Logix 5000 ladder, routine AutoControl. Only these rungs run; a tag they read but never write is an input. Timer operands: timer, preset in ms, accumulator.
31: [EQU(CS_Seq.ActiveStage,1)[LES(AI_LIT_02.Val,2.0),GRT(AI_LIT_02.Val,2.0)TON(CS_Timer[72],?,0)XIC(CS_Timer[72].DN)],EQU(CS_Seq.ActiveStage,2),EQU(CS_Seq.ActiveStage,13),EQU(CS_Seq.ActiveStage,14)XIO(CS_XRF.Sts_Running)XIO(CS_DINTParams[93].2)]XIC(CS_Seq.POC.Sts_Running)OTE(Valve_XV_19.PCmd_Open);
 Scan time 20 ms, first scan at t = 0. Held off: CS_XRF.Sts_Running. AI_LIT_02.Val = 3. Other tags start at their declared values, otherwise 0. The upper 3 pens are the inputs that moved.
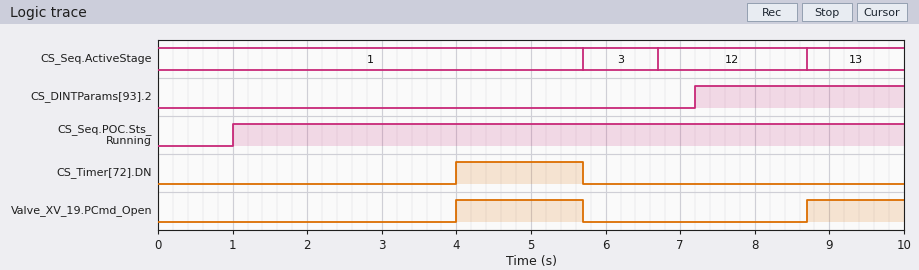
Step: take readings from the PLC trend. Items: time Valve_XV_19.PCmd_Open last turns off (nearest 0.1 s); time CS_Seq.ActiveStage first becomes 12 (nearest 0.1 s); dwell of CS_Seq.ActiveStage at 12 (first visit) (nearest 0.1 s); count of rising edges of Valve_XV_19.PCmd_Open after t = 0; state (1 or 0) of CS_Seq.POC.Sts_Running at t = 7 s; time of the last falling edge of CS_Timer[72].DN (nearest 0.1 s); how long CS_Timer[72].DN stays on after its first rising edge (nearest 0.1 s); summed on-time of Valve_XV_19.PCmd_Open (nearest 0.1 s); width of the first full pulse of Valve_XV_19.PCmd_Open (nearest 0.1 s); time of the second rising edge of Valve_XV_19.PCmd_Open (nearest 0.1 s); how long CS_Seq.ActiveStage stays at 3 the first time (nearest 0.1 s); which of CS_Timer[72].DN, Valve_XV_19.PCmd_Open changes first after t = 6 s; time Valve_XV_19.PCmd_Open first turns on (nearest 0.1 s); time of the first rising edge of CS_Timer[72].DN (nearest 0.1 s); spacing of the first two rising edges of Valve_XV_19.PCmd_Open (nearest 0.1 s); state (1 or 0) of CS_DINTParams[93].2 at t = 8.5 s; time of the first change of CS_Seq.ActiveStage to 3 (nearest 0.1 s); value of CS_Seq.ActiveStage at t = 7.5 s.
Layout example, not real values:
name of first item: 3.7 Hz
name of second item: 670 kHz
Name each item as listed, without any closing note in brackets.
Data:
time Valve_XV_19.PCmd_Open last turns off: 5.7 s
time CS_Seq.ActiveStage first becomes 12: 6.7 s
dwell of CS_Seq.ActiveStage at 12 (first visit): 2.0 s
count of rising edges of Valve_XV_19.PCmd_Open after t = 0: 2
state (1 or 0) of CS_Seq.POC.Sts_Running at t = 7 s: 1
time of the last falling edge of CS_Timer[72].DN: 5.7 s
how long CS_Timer[72].DN stays on after its first rising edge: 1.7 s
summed on-time of Valve_XV_19.PCmd_Open: 3.0 s
width of the first full pulse of Valve_XV_19.PCmd_Open: 1.7 s
time of the second rising edge of Valve_XV_19.PCmd_Open: 8.7 s
how long CS_Seq.ActiveStage stays at 3 the first time: 1.0 s
which of CS_Timer[72].DN, Valve_XV_19.PCmd_Open changes first after t = 6 s: Valve_XV_19.PCmd_Open
time Valve_XV_19.PCmd_Open first turns on: 4.0 s
time of the first rising edge of CS_Timer[72].DN: 4.0 s
spacing of the first two rising edges of Valve_XV_19.PCmd_Open: 4.7 s
state (1 or 0) of CS_DINTParams[93].2 at t = 8.5 s: 1
time of the first change of CS_Seq.ActiveStage to 3: 5.7 s
value of CS_Seq.ActiveStage at t = 7.5 s: 12
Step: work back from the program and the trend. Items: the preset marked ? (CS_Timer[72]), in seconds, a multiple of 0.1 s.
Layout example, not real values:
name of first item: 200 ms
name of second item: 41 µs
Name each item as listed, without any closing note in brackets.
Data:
the preset marked ? (CS_Timer[72]), in seconds, a multiple of 0.1 s: 4.0 s
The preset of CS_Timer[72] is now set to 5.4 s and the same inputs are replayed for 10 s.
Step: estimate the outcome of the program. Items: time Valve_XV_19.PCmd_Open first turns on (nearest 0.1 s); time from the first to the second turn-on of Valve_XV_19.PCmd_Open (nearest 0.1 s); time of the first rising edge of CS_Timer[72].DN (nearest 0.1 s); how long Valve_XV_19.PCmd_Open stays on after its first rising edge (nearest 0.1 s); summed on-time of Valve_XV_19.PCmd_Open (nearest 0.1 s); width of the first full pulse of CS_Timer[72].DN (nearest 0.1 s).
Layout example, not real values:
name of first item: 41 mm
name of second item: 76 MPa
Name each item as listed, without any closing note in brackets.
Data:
time Valve_XV_19.PCmd_Open first turns on: 5.4 s
time from the first to the second turn-on of Valve_XV_19.PCmd_Open: 3.3 s
time of the first rising edge of CS_Timer[72].DN: 5.4 s
how long Valve_XV_19.PCmd_Open stays on after its first rising edge: 0.3 s
summed on-time of Valve_XV_19.PCmd_Open: 1.6 s
width of the first full pulse of CS_Timer[72].DN: 0.3 s
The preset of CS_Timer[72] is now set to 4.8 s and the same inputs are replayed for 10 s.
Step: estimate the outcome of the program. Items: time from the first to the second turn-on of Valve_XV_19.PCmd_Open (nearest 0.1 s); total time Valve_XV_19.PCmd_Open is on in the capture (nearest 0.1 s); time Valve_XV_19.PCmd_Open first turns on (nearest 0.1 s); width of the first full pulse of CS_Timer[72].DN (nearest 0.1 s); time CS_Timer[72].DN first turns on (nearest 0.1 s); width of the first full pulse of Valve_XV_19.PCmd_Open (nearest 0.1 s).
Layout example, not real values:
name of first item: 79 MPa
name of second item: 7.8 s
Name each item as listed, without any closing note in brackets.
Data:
time from the first to the second turn-on of Valve_XV_19.PCmd_Open: 3.9 s
total time Valve_XV_19.PCmd_Open is on in the capture: 2.2 s
time Valve_XV_19.PCmd_Open first turns on: 4.8 s
width of the first full pulse of CS_Timer[72].DN: 0.9 s
time CS_Timer[72].DN first turns on: 4.8 s
width of the first full pulse of Valve_XV_19.PCmd_Open: 0.9 s
